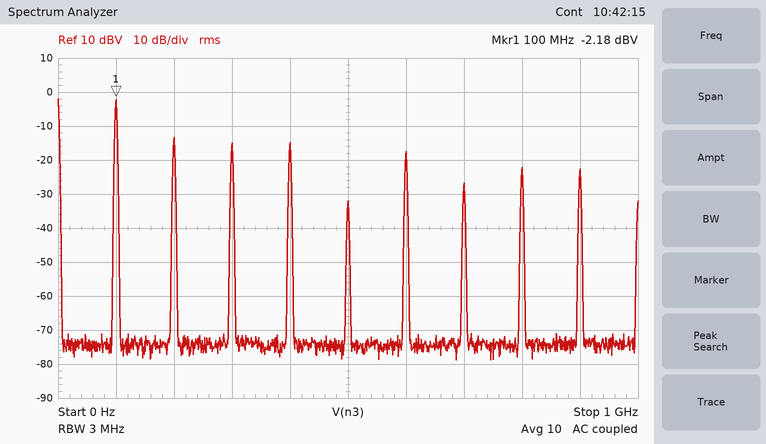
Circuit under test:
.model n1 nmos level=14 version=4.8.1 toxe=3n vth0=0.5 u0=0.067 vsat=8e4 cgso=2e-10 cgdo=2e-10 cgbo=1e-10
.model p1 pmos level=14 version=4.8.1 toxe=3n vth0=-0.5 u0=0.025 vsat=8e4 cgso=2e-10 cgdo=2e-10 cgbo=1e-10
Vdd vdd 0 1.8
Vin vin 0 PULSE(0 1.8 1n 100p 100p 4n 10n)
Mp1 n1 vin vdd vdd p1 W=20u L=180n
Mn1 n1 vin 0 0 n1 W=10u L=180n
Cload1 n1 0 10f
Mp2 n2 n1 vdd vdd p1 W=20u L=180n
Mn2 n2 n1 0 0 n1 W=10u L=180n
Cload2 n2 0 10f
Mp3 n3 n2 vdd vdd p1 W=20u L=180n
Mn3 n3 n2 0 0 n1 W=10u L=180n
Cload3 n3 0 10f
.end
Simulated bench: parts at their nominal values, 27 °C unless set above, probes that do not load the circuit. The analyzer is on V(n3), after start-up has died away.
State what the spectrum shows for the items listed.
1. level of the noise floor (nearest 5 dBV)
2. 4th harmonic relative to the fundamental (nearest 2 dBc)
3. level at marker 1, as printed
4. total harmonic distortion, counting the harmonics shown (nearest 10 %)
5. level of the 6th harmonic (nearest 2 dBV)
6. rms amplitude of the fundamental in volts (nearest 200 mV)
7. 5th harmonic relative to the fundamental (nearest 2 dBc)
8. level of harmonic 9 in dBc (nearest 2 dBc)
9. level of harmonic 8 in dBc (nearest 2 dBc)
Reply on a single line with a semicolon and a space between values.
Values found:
-75 dBV; -12 dBc; -2.18 dBV; 50 %; -18 dBV; 800 mV; -30 dBc; -20 dBc; -20 dBc
